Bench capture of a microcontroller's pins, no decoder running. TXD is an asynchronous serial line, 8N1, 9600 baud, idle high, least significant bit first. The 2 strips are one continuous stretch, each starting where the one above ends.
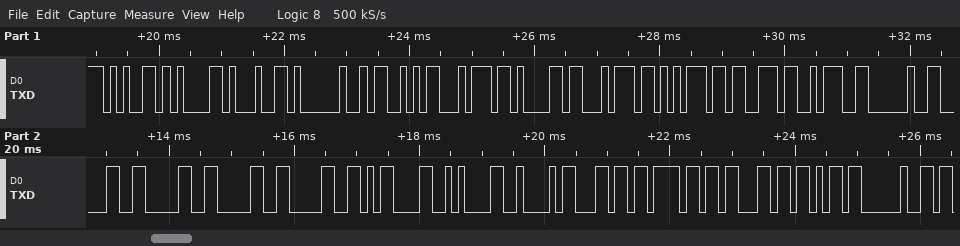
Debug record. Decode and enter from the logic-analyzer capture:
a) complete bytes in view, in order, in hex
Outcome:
65 61 64 20 53 74 61 74 75 73 3A 20 30 30 30 30 0D 0A 42 6C 6F 63 6B 20
